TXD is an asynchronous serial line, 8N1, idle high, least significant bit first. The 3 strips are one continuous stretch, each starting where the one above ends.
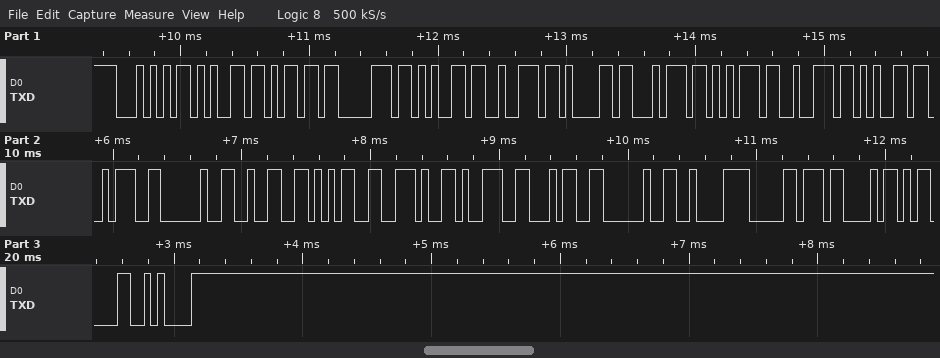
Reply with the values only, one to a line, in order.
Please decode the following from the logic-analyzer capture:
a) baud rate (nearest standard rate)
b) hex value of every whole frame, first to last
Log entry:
19200 baud
54 65 6D 70 65 72 61 74 75 72 65 3A 20 32 35 2E 39 34 20 C2 B0 43 0D 0A
